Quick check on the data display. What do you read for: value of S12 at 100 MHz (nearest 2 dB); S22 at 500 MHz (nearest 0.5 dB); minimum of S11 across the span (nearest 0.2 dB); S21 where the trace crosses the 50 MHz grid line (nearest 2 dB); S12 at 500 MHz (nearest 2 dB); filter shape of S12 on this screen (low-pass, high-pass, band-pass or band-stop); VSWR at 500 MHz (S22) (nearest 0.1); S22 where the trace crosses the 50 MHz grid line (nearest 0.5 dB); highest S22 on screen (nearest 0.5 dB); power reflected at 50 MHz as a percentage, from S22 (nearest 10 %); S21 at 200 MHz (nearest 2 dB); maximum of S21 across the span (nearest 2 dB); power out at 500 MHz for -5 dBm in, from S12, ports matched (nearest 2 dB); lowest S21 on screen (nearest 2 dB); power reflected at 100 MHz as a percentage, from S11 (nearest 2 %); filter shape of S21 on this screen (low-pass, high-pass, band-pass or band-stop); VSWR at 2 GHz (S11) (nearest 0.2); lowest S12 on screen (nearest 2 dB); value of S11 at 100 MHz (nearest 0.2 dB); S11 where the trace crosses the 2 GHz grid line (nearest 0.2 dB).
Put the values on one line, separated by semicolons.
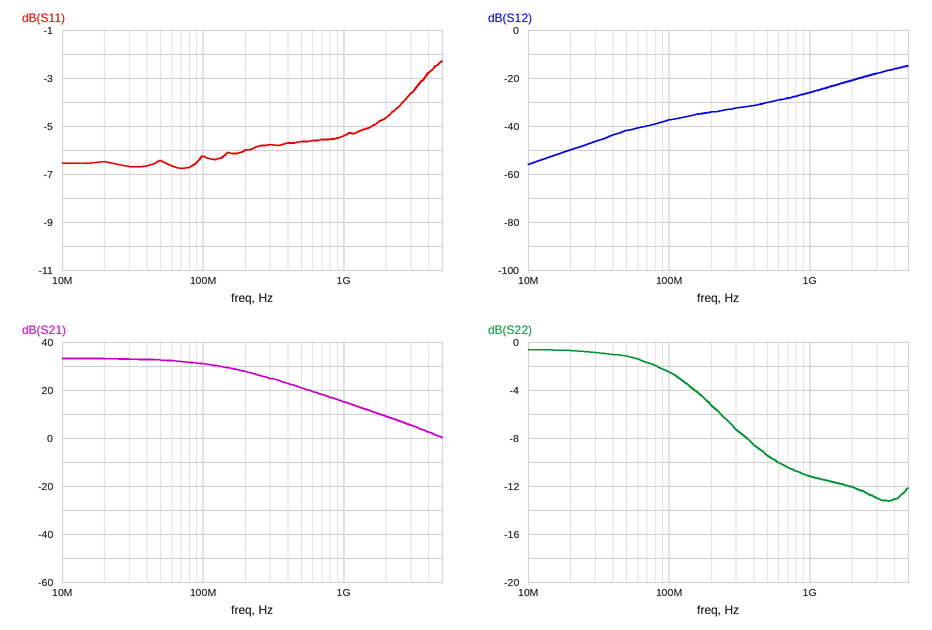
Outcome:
-38 dB; -9.5 dB; -6.8 dB; 32 dB; -30 dB; high-pass; 2.0; -1.0 dB; -0.5 dB; 80 %; 28 dB; 34 dB; -36 dBm; 0 dB; 24 %; low-pass; 3.8; -56 dB; -6.2 dB; -4.6 dB
